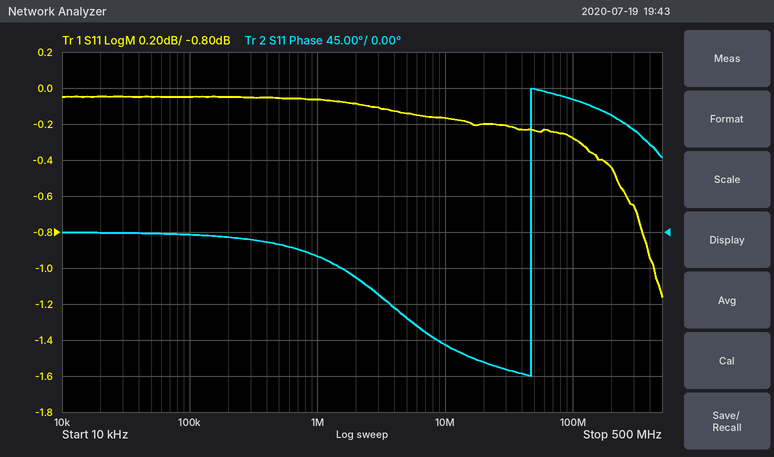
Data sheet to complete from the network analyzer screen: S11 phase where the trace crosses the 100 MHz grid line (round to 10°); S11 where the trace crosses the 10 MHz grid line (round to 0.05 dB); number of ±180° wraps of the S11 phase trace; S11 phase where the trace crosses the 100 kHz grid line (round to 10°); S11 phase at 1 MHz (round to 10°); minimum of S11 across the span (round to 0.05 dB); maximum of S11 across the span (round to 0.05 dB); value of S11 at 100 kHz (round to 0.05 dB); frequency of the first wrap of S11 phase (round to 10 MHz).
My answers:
170°
-0.15 dB
1
0°
-30°
-1.15 dB
-0.05 dB
-0.05 dB
50 MHz
